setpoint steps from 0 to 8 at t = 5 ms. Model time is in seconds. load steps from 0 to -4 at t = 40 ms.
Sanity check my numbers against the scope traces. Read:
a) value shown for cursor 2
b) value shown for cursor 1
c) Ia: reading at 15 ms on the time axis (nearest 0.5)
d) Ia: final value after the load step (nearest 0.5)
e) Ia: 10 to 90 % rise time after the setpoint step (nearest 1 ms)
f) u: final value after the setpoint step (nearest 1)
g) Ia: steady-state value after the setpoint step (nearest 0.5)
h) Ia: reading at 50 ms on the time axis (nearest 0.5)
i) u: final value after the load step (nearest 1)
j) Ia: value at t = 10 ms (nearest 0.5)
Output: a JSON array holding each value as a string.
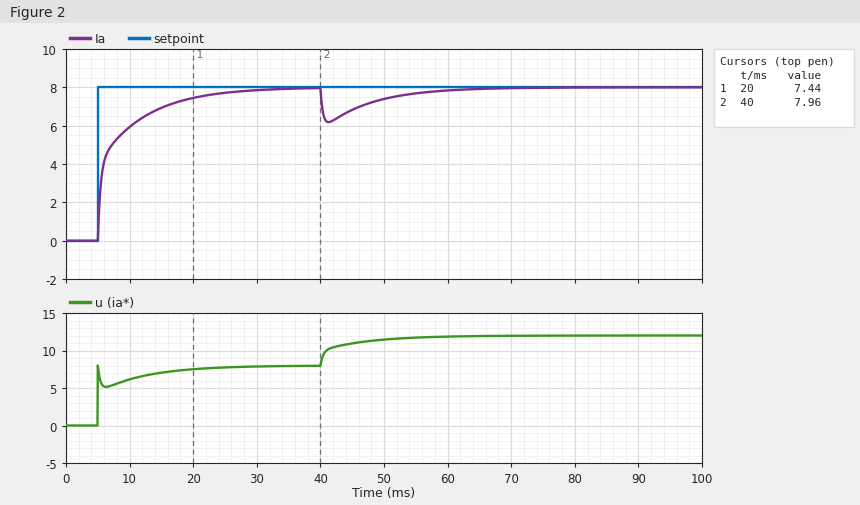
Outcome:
["7.96", "7.44", "7.0", "8.0", "12 ms", "8", "8.0", "7.5", "12", "6.0"]
